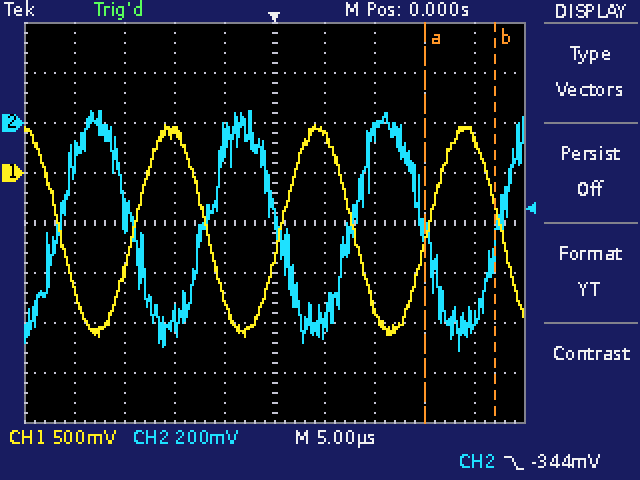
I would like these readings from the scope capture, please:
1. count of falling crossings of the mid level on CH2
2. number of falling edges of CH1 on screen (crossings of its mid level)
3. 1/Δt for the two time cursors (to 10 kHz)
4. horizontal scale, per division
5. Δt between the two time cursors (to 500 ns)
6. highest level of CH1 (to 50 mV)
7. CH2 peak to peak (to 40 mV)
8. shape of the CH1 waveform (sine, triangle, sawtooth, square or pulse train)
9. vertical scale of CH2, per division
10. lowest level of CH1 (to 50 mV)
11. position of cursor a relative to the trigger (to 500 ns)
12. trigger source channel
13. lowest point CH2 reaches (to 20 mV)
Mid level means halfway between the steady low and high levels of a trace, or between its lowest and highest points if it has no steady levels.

3
4
140 kHz
5 µs
7.0 µs
500 mV
960 mV
sine
200 mV
-1.65 V
+15.0 µs
CH2
-920 mV
